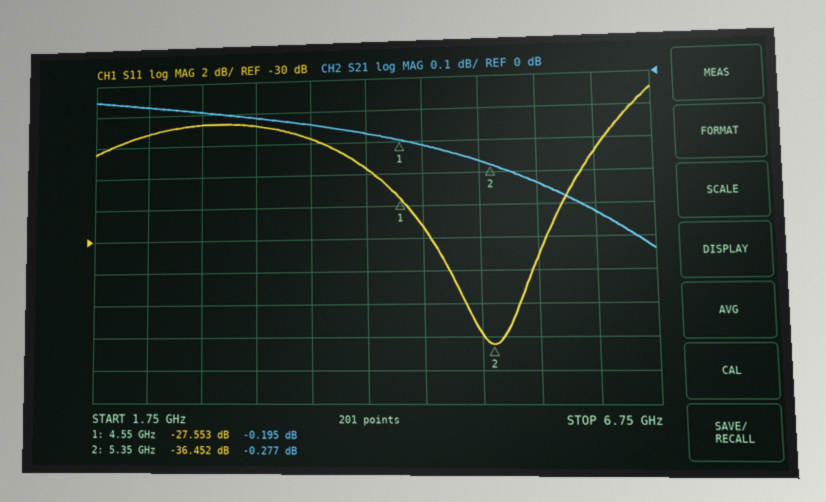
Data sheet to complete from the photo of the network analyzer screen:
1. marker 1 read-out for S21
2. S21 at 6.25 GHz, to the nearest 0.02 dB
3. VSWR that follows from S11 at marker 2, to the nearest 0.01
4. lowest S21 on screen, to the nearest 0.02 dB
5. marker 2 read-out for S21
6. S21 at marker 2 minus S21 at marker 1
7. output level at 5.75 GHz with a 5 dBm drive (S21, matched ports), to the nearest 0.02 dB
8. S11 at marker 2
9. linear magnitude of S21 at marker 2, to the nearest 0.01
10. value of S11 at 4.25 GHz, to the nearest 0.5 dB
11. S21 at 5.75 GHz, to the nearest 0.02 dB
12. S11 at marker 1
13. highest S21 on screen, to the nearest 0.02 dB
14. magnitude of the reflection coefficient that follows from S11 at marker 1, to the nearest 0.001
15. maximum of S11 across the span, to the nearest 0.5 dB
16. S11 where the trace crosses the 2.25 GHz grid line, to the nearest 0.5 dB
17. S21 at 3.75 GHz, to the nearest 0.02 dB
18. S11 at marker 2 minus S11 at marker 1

-0.195 dB
-0.42 dB
1.03
-0.54 dB
-0.277 dB
-0.082 dB
4.66 dBm
-36.452 dB
0.97
-25.5 dB
-0.34 dB
-27.553 dB
-0.06 dB
0.042
-21.0 dB
-23.0 dB
-0.14 dB
-8.899 dB
